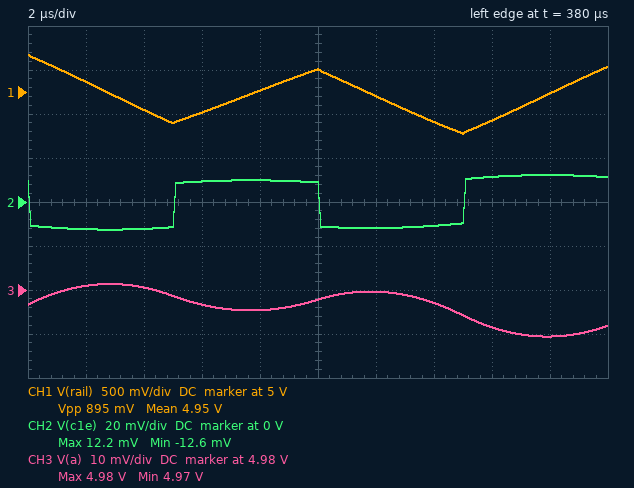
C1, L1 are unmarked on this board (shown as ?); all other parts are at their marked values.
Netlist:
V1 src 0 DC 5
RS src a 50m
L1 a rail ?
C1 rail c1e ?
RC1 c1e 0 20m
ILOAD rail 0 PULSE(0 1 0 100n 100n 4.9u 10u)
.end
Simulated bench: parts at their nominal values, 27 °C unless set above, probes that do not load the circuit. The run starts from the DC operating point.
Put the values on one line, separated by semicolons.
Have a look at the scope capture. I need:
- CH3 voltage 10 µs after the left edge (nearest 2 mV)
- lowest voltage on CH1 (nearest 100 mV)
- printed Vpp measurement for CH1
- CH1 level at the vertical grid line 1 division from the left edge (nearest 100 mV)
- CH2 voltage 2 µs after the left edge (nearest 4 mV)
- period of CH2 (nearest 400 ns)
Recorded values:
4.978 V; 4.5 V; 895 mV; 5.1 V; -12 mV; 10.0 µs
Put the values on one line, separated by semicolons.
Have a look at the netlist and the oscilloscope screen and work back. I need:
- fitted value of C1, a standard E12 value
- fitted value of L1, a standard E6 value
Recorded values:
3.9 µF; 6.8 µH
